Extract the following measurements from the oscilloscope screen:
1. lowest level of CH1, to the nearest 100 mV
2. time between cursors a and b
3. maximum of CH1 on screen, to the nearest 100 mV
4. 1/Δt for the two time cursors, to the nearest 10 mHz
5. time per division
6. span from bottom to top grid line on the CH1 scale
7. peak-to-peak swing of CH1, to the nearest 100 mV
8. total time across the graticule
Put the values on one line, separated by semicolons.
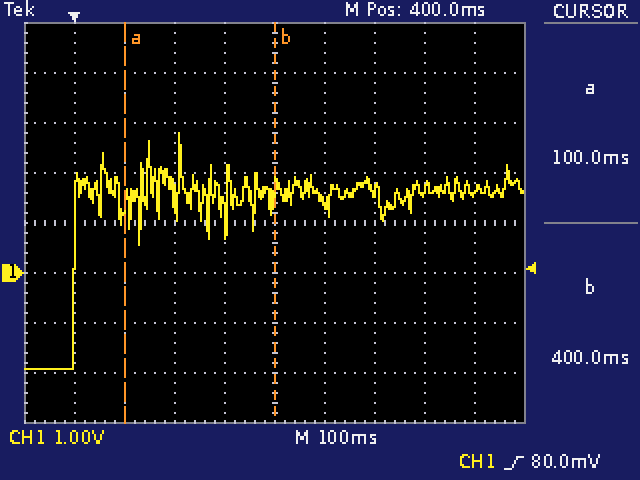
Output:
-1.9 V; 300 ms; 2.8 V; 3.33 Hz; 100 ms; 8 V; 4.7 V; 1 s
